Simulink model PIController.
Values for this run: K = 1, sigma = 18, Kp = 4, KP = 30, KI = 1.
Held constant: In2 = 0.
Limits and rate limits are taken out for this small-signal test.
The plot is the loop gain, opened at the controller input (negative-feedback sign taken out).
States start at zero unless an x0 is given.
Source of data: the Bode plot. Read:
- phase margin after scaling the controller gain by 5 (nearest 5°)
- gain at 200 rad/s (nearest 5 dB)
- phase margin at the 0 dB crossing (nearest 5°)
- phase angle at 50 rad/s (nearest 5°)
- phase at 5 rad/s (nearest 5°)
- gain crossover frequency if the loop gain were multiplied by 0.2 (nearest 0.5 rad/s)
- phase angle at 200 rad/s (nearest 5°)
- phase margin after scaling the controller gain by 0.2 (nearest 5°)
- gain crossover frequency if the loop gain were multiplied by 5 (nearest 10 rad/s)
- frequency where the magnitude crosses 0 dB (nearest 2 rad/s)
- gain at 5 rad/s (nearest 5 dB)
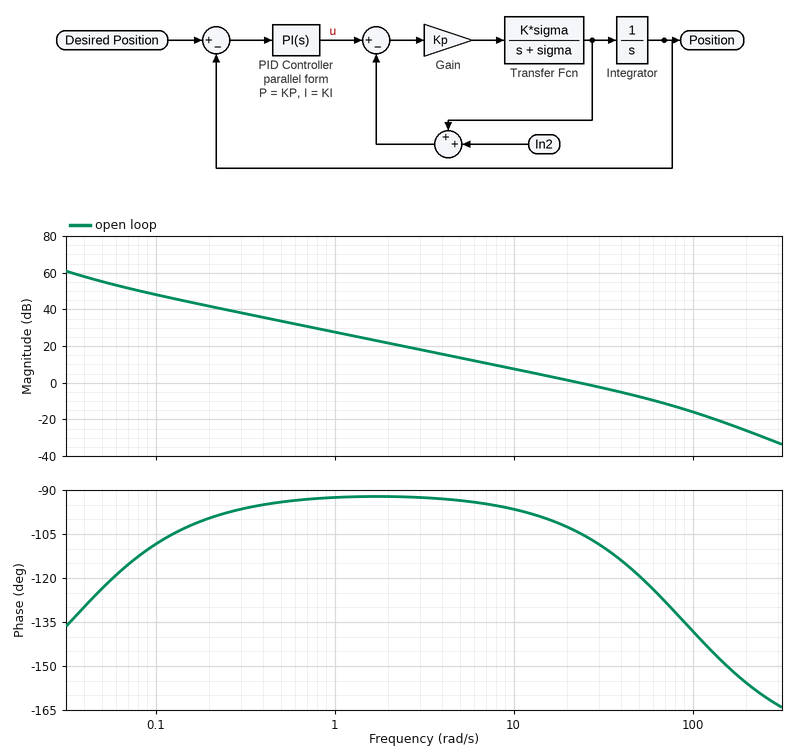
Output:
45°
-25 dB
75°
-120°
-95°
5.0 rad/s
-155°
85°
90 rad/s
24 rad/s
15 dB
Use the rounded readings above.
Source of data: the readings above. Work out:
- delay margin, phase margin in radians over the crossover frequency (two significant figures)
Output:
0.055 s
